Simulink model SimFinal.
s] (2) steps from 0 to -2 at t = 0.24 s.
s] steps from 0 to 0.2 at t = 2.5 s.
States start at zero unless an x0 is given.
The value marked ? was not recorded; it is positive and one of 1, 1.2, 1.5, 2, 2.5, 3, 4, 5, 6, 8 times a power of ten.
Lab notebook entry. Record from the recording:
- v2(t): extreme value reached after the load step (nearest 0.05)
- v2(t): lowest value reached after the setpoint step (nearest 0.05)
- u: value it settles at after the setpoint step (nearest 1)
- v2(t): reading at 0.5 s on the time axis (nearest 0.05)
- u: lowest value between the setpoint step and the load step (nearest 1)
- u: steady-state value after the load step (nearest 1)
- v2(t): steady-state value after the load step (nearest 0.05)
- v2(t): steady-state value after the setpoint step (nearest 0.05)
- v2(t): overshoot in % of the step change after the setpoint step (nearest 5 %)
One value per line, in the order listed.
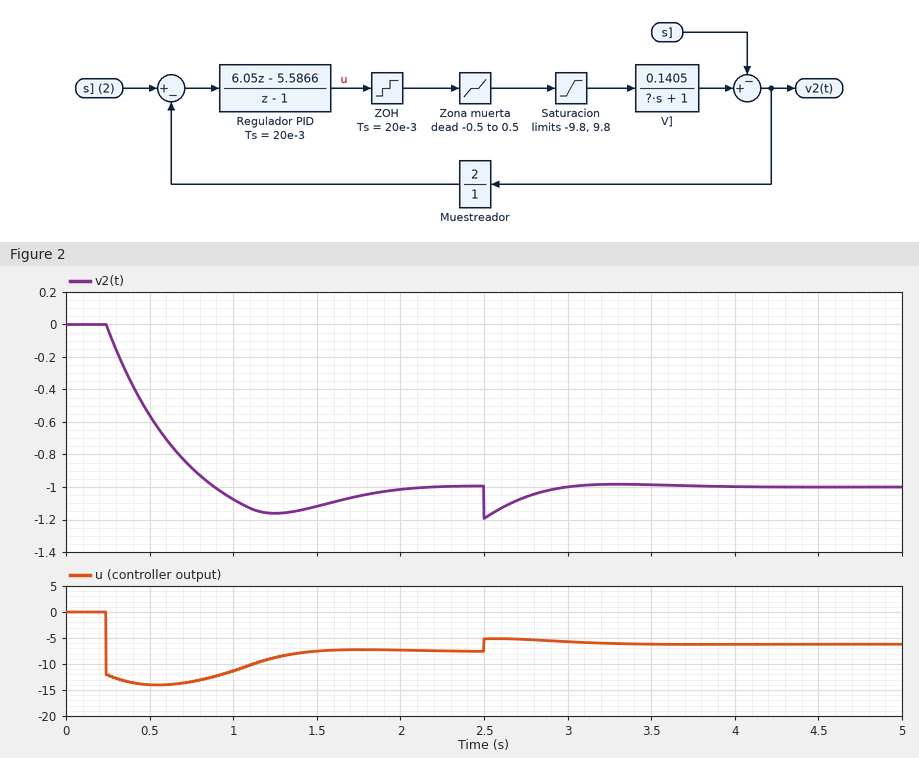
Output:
-1.20
-1.15
-8
-0.55
-14
-6
-1.00
-1.00
15 %
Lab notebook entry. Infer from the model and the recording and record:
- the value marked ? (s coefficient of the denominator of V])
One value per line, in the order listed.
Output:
0.5
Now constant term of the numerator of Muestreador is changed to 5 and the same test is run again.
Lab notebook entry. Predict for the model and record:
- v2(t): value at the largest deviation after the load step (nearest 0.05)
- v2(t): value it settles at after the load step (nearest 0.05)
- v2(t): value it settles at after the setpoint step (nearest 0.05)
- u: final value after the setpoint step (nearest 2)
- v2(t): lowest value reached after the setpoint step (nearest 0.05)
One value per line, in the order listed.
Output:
-0.60
-0.40
-0.40
-4
-0.45
